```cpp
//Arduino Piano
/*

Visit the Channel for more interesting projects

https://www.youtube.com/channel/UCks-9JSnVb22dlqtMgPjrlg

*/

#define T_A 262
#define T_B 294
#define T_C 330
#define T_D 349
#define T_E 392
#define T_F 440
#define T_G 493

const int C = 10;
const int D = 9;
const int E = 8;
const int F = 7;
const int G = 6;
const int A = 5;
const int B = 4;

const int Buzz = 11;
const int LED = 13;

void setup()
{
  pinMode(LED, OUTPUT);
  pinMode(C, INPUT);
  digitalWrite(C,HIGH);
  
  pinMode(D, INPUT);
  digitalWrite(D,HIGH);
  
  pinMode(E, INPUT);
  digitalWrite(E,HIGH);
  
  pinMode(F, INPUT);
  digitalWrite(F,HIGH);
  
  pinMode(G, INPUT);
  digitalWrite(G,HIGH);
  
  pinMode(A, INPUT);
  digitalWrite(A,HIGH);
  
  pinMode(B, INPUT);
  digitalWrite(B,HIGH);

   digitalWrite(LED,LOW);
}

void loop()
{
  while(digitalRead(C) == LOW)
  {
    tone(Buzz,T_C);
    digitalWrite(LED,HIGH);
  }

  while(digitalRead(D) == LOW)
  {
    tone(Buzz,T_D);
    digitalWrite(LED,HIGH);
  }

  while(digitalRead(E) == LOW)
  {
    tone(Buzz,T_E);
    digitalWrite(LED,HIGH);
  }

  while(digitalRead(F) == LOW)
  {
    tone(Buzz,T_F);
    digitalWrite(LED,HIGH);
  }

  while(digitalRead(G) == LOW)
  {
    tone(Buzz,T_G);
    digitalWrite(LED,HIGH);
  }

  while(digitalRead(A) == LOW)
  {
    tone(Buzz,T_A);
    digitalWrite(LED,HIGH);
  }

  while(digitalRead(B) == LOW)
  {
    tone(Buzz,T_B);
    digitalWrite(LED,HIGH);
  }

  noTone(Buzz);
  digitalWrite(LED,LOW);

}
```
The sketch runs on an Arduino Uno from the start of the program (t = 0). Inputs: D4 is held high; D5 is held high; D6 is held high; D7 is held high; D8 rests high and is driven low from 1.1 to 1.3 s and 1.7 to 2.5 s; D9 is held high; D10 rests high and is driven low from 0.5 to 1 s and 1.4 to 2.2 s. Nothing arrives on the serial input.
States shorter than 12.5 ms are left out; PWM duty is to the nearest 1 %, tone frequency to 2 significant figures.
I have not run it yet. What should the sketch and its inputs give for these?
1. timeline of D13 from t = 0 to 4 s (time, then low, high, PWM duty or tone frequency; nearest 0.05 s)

0 s low; 0.5 s high; 1 s low; 1.1 s high; 1.3 s low; 1.4 s high; 2.5 s low
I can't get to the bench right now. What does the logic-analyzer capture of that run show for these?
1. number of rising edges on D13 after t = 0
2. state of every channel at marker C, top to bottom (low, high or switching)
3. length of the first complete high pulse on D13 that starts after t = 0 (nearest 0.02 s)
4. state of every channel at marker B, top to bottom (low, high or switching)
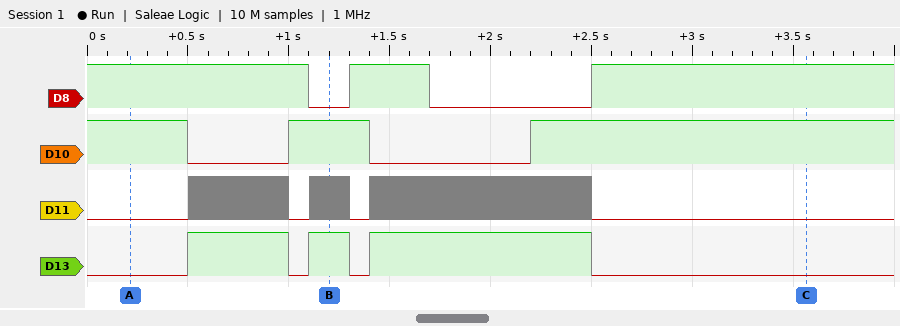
3
D8 high, D10 high, D11 low, D13 low
0.50 s
D8 low, D10 high, D11 switching, D13 high
